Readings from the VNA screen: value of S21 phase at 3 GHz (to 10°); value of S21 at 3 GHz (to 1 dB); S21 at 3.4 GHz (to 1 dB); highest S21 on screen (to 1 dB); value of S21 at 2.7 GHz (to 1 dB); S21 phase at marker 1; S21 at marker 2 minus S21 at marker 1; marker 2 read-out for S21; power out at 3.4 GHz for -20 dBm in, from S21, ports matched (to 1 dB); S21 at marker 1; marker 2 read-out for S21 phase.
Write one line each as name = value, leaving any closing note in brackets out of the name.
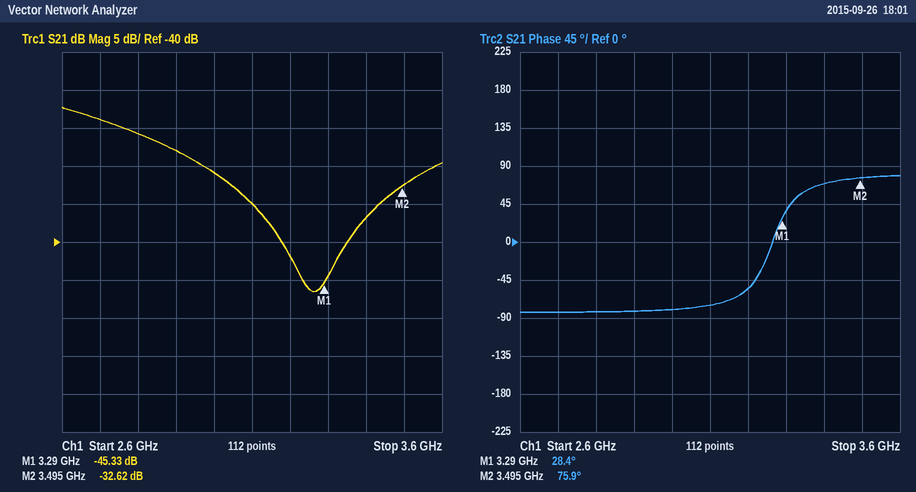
value of S21 phase at 3 GHz = -80°
value of S21 at 3 GHz = -31 dB
S21 at 3.4 GHz = -37 dB
highest S21 on screen = -22 dB
value of S21 at 2.7 GHz = -24 dB
S21 phase at marker 1 = 28.4°
S21 at marker 2 minus S21 at marker 1 = 12.71 dB
marker 2 read-out for S21 = -32.62 dB
power out at 3.4 GHz for -20 dBm in, from S21, ports matched = -57 dBm
S21 at marker 1 = -45.33 dB
marker 2 read-out for S21 phase = 75.9°
